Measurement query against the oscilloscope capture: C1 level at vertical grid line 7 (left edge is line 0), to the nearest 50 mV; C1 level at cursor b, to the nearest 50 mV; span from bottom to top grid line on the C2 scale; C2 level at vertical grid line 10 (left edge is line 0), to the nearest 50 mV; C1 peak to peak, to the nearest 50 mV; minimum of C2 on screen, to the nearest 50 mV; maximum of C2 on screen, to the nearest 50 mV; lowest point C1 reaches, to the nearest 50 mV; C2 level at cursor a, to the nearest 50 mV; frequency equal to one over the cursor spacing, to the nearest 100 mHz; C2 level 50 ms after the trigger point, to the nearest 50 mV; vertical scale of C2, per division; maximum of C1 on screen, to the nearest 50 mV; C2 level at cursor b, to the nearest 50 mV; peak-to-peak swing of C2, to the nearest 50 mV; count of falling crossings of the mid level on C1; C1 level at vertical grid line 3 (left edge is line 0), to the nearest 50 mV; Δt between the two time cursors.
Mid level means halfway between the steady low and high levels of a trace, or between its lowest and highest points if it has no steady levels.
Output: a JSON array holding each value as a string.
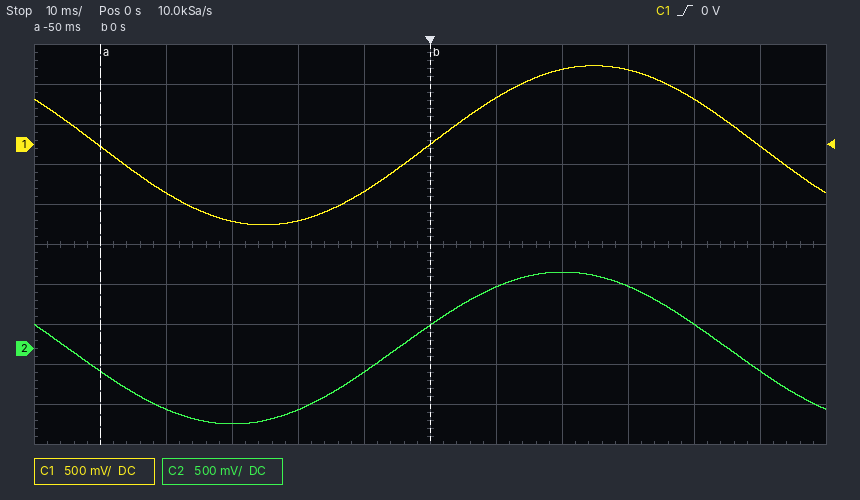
["600 mV", "0 mV", "5 V", "300 mV", "2.00 V", "-950 mV", "950 mV", "-1.00 V", "-300 mV", "20.0 Hz", "-300 mV", "500 mV", "1.00 V", "300 mV", "1.90 V", "2", "-950 mV", "50 ms"]
